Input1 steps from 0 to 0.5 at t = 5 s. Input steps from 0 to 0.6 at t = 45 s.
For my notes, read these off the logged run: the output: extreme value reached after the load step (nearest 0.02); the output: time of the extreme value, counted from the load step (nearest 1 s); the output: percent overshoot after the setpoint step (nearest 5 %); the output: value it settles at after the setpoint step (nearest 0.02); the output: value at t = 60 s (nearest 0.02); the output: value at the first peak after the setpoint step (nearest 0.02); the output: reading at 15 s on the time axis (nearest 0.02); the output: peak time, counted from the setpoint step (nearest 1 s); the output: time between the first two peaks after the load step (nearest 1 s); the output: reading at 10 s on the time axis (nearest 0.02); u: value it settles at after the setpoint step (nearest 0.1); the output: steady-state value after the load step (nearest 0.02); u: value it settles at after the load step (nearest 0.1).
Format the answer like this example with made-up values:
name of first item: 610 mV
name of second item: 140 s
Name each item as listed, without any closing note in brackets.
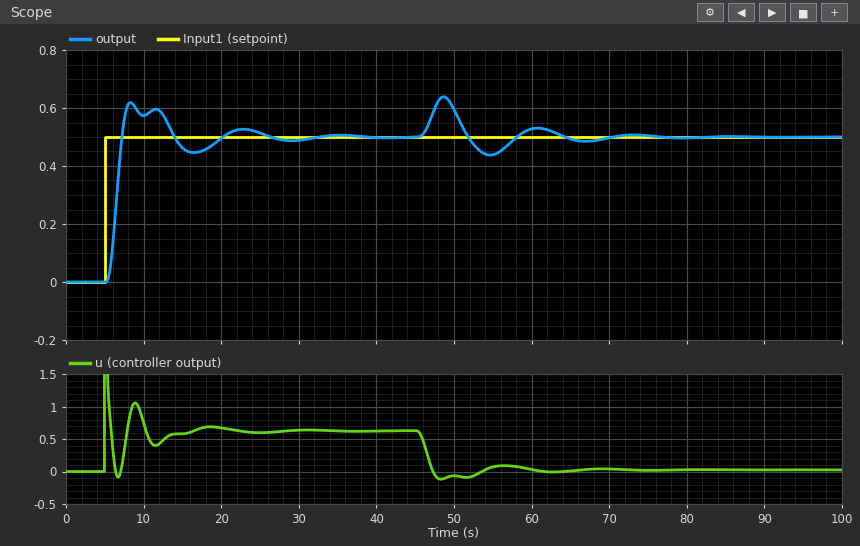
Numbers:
the output: extreme value reached after the load step: 0.64
the output: time of the extreme value, counted from the load step: 4 s
the output: percent overshoot after the setpoint step: 25 %
the output: value it settles at after the setpoint step: 0.50
the output: value at t = 60 s: 0.52
the output: value at the first peak after the setpoint step: 0.62
the output: reading at 15 s on the time axis: 0.46
the output: peak time, counted from the setpoint step: 3 s
the output: time between the first two peaks after the load step: 12 s
the output: reading at 10 s on the time axis: 0.58
u: value it settles at after the setpoint step: 0.6
the output: steady-state value after the load step: 0.50
u: value it settles at after the load step: 0.0
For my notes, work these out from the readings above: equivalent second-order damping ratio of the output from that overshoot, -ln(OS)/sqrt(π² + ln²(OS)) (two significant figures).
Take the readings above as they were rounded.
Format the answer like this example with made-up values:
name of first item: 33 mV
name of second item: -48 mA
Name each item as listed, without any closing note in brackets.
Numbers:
equivalent second-order damping ratio of the output from that overshoot, -ln(OS)/sqrt(π² + ln²(OS)): 0.40
